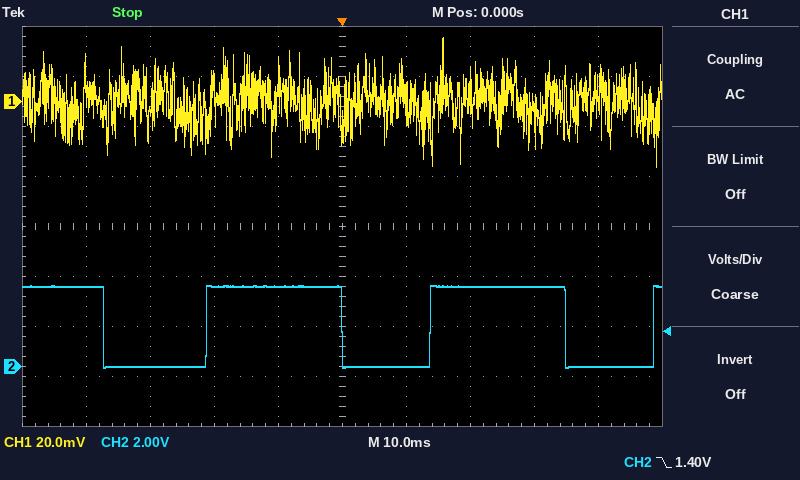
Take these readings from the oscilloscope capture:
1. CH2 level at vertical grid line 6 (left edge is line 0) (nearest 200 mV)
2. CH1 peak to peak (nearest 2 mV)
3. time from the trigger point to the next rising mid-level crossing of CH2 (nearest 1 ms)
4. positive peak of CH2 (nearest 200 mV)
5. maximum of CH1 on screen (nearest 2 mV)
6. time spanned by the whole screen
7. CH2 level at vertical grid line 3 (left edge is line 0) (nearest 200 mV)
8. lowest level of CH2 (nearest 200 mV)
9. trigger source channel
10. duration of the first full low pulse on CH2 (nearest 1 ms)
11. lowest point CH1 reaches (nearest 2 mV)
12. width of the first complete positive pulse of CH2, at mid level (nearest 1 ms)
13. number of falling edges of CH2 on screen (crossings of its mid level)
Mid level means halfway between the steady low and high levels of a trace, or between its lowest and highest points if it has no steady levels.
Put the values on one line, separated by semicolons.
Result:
0.0 V; 52 mV; 14 ms; 3.2 V; 26 mV; 100 ms; 3.2 V; 0.0 V; CH2; 16 ms; -26 mV; 21 ms; 3
